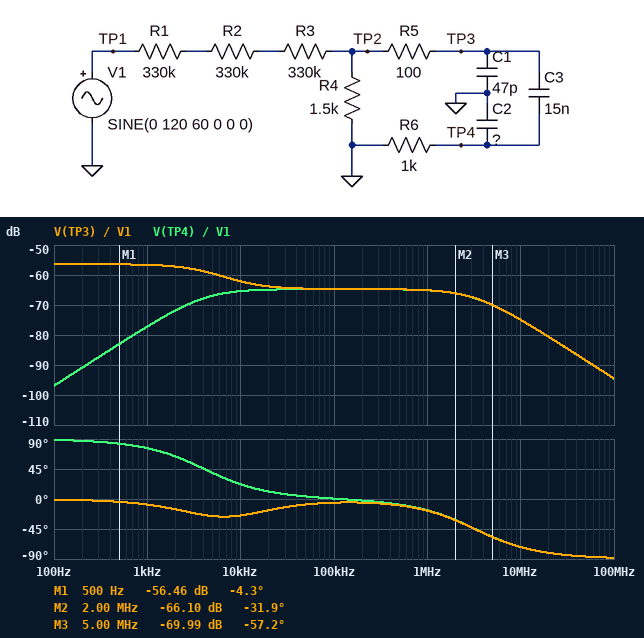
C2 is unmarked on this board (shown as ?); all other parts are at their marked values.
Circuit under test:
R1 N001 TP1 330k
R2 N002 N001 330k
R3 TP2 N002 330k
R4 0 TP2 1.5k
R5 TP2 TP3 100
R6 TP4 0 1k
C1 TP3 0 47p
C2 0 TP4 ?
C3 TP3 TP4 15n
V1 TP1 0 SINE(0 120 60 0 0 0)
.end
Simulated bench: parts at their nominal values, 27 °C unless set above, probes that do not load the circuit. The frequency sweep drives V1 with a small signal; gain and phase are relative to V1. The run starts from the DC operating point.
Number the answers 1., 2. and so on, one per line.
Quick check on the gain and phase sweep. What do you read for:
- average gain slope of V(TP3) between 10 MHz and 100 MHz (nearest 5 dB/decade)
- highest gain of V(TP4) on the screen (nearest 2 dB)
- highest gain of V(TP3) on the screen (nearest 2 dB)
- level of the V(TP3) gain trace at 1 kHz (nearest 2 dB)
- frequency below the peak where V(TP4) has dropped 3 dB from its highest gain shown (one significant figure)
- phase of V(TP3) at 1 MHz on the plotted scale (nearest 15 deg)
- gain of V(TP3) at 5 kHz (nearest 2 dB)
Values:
1. -20 dB/decade
2. -64 dB
3. -56 dB
4. -56 dB
5. 4 kHz
6. -15 deg
7. -60 dB
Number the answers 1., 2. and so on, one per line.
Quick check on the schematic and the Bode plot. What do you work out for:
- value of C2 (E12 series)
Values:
1. 33 pF
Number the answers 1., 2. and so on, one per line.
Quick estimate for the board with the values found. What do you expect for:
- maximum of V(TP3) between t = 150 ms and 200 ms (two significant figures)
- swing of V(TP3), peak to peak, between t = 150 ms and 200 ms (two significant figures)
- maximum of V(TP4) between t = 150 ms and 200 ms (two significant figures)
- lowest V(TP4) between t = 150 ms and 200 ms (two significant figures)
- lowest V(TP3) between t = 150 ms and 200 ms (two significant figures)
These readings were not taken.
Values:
1. 180 mV
2. 360 mV
3. 1.0 mV
4. -1.0 mV
5. -180 mV
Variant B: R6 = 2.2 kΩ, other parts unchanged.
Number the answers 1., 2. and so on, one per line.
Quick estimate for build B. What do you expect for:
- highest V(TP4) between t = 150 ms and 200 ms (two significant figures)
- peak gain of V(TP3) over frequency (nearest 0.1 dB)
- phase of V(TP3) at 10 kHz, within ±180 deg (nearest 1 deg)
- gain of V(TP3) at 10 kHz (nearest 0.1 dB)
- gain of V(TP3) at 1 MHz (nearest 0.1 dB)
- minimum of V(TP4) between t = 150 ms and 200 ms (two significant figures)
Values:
1. 2.3 mV
2. -56.4 dB
3. -10 deg
4. -60.6 dB
5. -62.0 dB
6. -2.3 mV
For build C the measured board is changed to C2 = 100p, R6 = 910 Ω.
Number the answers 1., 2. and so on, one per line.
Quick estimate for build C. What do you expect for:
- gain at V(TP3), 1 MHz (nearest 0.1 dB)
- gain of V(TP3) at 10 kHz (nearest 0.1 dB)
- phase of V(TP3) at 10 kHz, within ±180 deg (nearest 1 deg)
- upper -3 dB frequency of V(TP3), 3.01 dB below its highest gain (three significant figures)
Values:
1. -66.3 dB
2. -62.2 dB
3. -27 deg
4. 4.93 kHz
